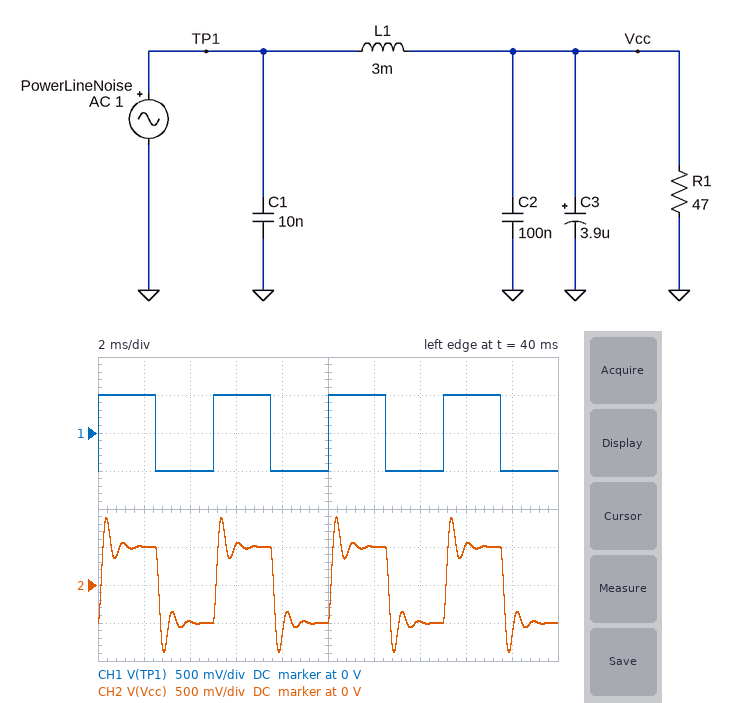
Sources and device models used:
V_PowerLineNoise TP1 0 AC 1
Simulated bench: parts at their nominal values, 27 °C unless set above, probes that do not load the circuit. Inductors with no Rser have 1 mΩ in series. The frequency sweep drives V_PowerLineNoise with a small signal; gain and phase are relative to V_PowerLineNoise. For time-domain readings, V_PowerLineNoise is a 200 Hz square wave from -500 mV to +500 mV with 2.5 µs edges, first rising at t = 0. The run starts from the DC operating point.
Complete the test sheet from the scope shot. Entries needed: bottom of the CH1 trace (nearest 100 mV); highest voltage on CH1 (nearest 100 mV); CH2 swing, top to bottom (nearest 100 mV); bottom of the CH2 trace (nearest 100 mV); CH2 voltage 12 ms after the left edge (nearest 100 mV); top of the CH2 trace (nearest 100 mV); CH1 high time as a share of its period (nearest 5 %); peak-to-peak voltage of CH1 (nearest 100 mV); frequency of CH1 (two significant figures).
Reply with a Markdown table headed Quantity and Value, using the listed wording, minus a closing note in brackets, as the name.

| Quantity | Value |
|---|---|
| bottom of the CH1 trace | -500 mV |
| highest voltage on CH1 | 500 mV |
| CH2 swing, top to bottom | 1.8 V |
| bottom of the CH2 trace | -900 mV |
| CH2 voltage 12 ms after the left edge | 500 mV |
| top of the CH2 trace | 900 mV |
| CH1 high time as a share of its period | 50 % |
| peak-to-peak voltage of CH1 | 1.0 V |
| frequency of CH1 | 200 Hz |
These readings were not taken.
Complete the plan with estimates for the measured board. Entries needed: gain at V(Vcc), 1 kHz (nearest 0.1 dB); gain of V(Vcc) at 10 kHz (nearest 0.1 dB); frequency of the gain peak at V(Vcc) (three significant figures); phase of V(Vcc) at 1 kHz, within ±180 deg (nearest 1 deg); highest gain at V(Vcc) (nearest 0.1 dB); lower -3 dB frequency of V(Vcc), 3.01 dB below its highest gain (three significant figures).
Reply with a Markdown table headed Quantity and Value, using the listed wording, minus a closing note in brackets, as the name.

| Quantity | Value |
|---|---|
| gain at V(Vcc), 1 kHz | 3.6 dB |
| gain of V(Vcc) at 10 kHz | -33.4 dB |
| frequency of the gain peak at V(Vcc) | 1.32 kHz |
| phase of V(Vcc) at 1 kHz, within ±180 deg | -37 deg |
| highest gain at V(Vcc) | 5.1 dB |
| lower -3 dB frequency of V(Vcc), 3.01 dB below its highest gain | 759 Hz |
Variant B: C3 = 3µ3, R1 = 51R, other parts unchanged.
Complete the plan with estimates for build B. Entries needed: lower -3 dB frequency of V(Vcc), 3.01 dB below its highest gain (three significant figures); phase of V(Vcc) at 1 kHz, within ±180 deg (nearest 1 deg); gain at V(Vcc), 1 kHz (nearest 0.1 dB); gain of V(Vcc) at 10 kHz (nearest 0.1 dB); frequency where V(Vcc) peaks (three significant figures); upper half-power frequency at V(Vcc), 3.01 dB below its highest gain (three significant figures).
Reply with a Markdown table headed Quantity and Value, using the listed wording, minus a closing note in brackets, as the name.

| Quantity | Value |
|---|---|
| lower -3 dB frequency of V(Vcc), 3.01 dB below its highest gain | 824 Hz |
| phase of V(Vcc) at 1 kHz, within ±180 deg | -32 deg |
| gain at V(Vcc), 1 kHz | 3.1 dB |
| gain of V(Vcc) at 10 kHz | -31.9 dB |
| frequency where V(Vcc) peaks | 1.44 kHz |
| upper half-power frequency at V(Vcc), 3.01 dB below its highest gain | 1.86 kHz |
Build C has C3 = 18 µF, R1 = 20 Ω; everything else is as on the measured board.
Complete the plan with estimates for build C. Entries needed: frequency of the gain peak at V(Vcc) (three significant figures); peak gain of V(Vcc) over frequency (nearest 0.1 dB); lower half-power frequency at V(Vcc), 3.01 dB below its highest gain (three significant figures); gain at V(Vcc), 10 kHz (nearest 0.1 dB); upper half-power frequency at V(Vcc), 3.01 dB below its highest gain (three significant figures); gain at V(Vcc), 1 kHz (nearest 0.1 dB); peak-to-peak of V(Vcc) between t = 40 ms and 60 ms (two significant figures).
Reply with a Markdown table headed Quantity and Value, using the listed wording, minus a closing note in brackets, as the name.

| Quantity | Value |
|---|---|
| frequency of the gain peak at V(Vcc) | 608 Hz |
| peak gain of V(Vcc) over frequency | 4.3 dB |
| lower half-power frequency at V(Vcc), 3.01 dB below its highest gain | 292 Hz |
| gain at V(Vcc), 10 kHz | -46.6 dB |
| upper half-power frequency at V(Vcc), 3.01 dB below its highest gain | 809 Hz |
| gain at V(Vcc), 1 kHz | -3.4 dB |
| peak-to-peak of V(Vcc) between t = 40 ms and 60 ms | 1.7 V |
